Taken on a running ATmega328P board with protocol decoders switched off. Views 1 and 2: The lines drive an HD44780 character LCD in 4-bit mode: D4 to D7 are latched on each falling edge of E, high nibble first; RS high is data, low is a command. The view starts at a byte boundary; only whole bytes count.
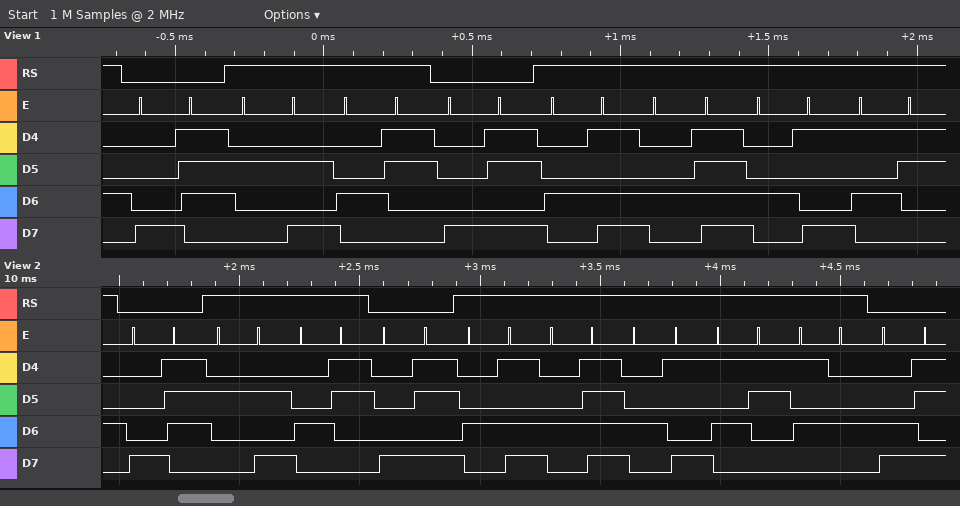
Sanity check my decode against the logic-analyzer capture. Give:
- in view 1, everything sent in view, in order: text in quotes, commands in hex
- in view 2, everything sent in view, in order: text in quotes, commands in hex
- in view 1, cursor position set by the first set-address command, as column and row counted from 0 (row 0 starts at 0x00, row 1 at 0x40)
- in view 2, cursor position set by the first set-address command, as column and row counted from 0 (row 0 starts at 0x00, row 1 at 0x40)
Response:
0x87 "*C" 0x8B "MOIS"
0x87 "*C" 0x8B "MOIST" 0xCB
column 7, row 0
column 7, row 0
